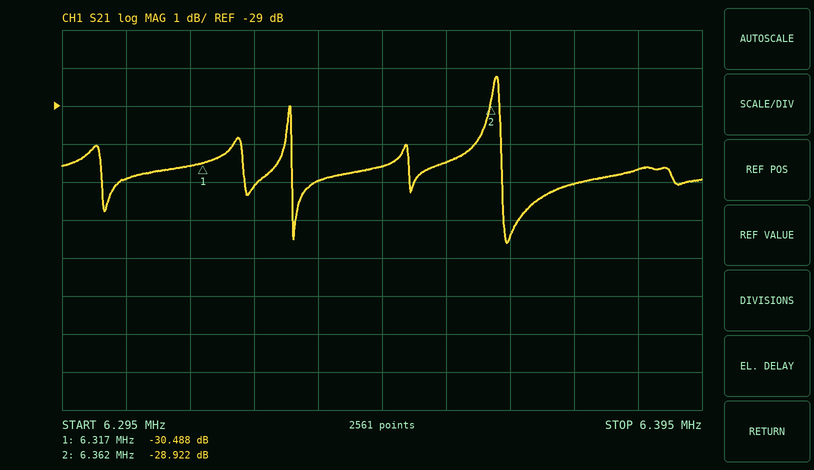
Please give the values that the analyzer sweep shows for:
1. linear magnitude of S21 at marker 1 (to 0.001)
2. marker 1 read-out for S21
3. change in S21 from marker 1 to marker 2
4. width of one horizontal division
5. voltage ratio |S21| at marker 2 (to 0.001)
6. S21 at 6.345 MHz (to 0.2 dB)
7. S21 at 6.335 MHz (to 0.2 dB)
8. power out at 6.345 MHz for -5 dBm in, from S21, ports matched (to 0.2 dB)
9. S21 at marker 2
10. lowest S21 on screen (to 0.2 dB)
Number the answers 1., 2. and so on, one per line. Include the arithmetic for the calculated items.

1. 10^(-30.488/20) ≈ 0.030
2. -30.488 dB
3. -28.922 − (-30.488) = 1.566 dB
4. 10 kHz
5. 10^(-28.922/20) ≈ 0.036
6. -30.6 dB
7. -31.0 dB
8. -5 dBm + (-30.6 dB) = -35.6 dBm
9. -28.922 dB
10. -32.6 dB
